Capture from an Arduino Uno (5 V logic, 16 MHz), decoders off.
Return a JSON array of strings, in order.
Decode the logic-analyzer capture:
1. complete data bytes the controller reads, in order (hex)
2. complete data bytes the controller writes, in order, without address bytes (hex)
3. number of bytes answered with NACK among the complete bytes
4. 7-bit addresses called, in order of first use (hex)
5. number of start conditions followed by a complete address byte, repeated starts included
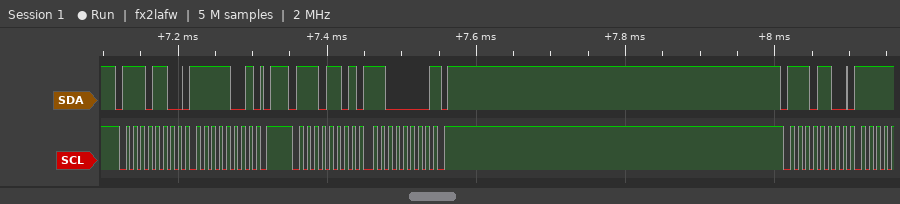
["C0", "F9", "1", "0x76", "3"]
